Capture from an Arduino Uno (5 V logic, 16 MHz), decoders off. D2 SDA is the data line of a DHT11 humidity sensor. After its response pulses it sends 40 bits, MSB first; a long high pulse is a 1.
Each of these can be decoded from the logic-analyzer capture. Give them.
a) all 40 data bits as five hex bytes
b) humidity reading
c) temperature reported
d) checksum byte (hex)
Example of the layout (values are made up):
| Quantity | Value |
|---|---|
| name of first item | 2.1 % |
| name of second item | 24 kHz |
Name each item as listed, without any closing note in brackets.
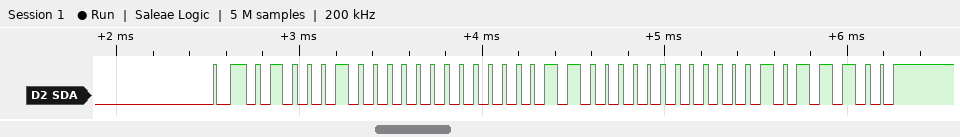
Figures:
| Quantity | Value |
|---|---|
| all 40 data bits as five hex bytes | 44 00 18 00 5C |
| humidity reading | 68 % |
| temperature reported | 24.0 °C |
| checksum byte | 0x5C |
